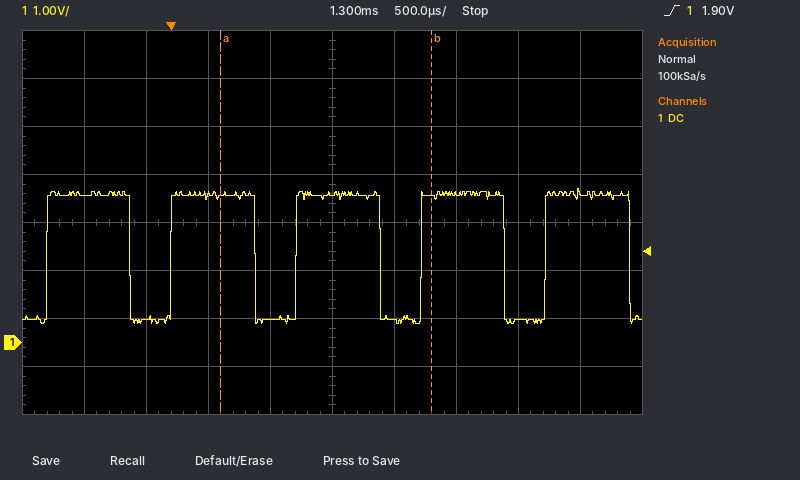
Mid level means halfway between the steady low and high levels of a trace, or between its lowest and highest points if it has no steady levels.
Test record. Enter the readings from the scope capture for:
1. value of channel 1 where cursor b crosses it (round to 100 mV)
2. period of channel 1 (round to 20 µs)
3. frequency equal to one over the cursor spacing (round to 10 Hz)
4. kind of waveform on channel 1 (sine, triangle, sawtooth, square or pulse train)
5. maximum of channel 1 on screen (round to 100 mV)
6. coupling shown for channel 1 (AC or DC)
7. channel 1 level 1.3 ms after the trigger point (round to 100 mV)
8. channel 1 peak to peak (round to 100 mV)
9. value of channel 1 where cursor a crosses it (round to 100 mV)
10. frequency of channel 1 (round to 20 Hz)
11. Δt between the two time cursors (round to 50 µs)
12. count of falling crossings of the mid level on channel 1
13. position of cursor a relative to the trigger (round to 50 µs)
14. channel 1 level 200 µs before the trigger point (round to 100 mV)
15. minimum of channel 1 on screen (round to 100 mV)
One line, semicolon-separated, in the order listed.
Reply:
3.0 V; 1.00 ms; 590 Hz; pulse train; 3.2 V; DC; 3.1 V; 2.8 V; 3.0 V; 1.00 kHz; 1.70 ms; 5; +400 µs; 500 mV; 400 mV
